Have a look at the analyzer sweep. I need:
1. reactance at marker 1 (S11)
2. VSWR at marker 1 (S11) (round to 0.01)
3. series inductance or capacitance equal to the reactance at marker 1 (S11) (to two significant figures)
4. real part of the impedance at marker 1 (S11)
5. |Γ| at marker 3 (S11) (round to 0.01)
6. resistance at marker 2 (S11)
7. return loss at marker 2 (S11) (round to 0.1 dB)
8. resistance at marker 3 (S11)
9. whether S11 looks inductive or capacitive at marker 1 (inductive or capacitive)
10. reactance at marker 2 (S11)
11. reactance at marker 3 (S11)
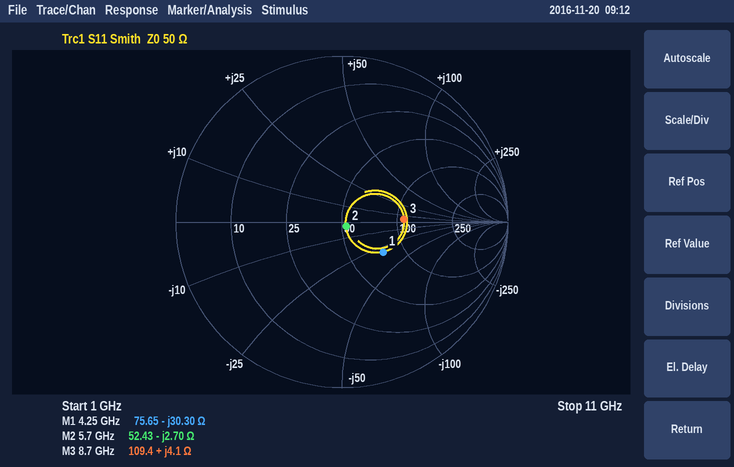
-30.30 Ω
1.89
1.2 pF
75.65 Ω
0.37
52.43 Ω
29.0 dB
109.4 Ω
capacitive
-2.70 Ω
+4.1 Ω
